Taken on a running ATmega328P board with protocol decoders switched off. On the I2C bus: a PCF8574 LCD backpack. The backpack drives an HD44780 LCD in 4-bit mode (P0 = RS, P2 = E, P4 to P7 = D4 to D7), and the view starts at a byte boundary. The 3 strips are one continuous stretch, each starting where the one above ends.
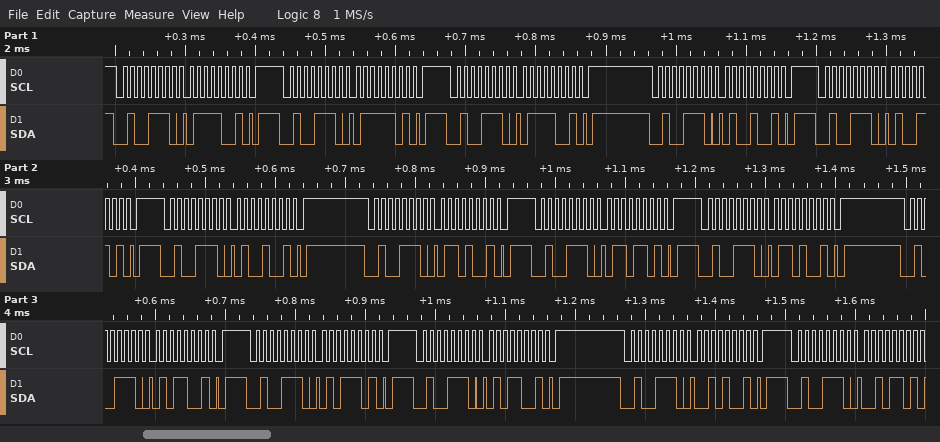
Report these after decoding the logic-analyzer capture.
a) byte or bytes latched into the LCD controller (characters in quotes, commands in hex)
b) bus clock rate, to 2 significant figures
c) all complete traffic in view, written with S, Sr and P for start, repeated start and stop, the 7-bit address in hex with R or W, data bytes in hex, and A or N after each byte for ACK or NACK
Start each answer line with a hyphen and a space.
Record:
- 't' 'e'
- 100 kHz
- S 27W A 79 A P S 27W A 7D A P S 27W A 79 A P S 27W A 49 A P S 27W A 4D A P S 27W A 49 A P S 27W A 69 A P S 27W A 6D A P S 27W A 69 A P S 27W A 59 A P S 27W A 5D A P S 27W A 59 A P S 27W A 29 A P S 27W A 2D A
